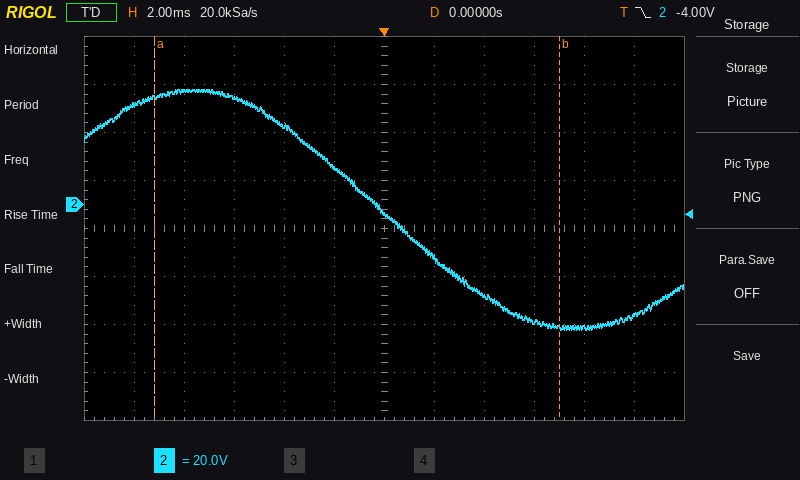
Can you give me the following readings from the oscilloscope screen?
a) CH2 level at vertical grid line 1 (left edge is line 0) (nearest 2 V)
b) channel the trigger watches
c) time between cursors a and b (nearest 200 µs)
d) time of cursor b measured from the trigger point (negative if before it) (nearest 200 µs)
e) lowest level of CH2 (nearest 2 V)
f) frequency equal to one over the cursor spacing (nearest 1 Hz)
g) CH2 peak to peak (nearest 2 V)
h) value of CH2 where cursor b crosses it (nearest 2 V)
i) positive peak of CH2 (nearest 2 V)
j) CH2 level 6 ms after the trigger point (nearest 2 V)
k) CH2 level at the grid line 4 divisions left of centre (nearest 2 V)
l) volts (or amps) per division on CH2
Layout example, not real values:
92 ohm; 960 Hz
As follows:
42 V; CH2; 16.2 ms; +7.0 ms; -52 V; 62 Hz; 100 V; -52 V; 48 V; -48 V; 48 V; 20 V
